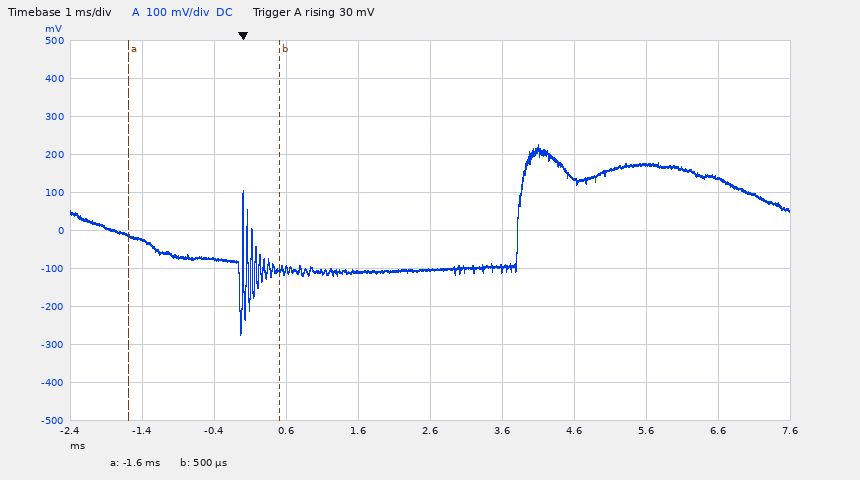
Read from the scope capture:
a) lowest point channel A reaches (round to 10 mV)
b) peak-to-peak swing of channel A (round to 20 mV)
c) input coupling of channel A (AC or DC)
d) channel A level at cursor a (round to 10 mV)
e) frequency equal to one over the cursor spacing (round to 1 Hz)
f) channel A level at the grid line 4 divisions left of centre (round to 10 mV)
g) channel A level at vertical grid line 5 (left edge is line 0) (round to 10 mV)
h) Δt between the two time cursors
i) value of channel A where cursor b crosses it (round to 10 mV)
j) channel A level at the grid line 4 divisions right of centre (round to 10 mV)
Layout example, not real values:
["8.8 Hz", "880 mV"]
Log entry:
["-270 mV", "500 mV", "DC", "-10 mV", "476 Hz", "-20 mV", "-100 mV", "2.1 ms", "-100 mV", "140 mV"]
